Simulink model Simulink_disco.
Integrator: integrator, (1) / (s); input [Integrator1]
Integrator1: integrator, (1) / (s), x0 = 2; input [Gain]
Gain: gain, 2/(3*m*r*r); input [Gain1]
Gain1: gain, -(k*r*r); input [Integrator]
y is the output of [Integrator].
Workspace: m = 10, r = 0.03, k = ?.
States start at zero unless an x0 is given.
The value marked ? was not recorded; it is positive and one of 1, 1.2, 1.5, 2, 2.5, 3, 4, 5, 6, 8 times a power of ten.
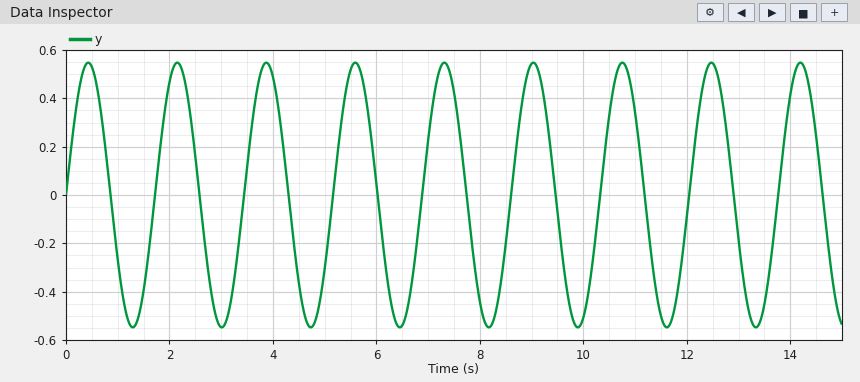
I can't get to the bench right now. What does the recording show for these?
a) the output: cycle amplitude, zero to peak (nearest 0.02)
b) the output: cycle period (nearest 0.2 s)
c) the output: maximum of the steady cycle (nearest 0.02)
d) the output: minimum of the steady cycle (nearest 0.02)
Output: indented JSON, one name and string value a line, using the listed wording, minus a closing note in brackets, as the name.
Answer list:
{
  "the output: cycle amplitude, zero to peak": "0.54",
  "the output: cycle period": "1.8 s",
  "the output: maximum of the steady cycle": "0.54",
  "the output: minimum of the steady cycle": "-0.54"
}
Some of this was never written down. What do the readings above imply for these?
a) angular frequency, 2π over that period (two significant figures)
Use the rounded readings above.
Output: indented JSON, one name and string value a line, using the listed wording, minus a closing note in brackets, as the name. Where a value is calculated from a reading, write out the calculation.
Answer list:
{
  "angular frequency, 2π over that period": "2π / 1.8 = 3.5 rad/s"
}
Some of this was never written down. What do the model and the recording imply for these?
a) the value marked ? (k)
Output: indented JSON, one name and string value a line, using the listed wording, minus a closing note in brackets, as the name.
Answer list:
{
  "the value marked ?": "200"
}
